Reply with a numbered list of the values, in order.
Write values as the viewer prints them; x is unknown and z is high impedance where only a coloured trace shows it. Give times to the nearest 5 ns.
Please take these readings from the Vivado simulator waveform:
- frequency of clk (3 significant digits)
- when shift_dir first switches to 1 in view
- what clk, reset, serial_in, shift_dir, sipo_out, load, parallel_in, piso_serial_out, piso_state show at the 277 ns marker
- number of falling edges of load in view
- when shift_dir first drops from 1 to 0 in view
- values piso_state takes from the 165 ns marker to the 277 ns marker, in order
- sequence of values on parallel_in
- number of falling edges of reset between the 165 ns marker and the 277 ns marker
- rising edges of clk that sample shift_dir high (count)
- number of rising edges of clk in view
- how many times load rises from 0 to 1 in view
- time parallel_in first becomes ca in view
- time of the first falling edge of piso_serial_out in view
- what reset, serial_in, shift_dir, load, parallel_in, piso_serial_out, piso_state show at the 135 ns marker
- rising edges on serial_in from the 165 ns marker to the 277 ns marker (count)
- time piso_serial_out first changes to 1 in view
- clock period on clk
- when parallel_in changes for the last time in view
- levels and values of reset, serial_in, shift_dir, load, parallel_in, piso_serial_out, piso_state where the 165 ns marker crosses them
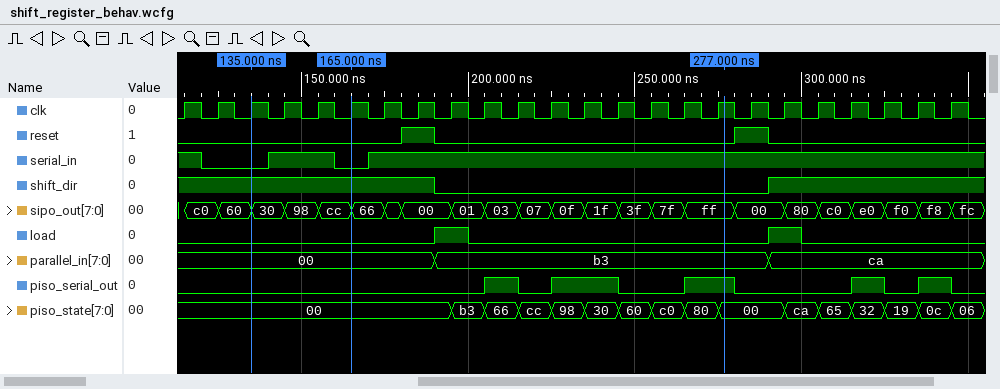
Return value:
1. 100 MHz
2. 290 ns
3. clk=1, reset=0, serial_in=1, shift_dir=0, sipo_out=ff, load=0, parallel_in=b3, piso_serial_out=1, piso_state=00
4. 2
5. 190 ns
6. 00, b3, 66, cc, 98, 30, 60, c0, 80, 00
7. 00, b3, ca
8. 1
9. 14
10. 24
11. 2
12. 290 ns
13. 215 ns
14. reset=0, serial_in=0, shift_dir=1, load=0, parallel_in=00, piso_serial_out=0, piso_state=00
15. 1
16. 205 ns
17. 10 ns
18. 290 ns
19. reset=0, serial_in=0, shift_dir=1, load=0, parallel_in=00, piso_serial_out=0, piso_state=00
